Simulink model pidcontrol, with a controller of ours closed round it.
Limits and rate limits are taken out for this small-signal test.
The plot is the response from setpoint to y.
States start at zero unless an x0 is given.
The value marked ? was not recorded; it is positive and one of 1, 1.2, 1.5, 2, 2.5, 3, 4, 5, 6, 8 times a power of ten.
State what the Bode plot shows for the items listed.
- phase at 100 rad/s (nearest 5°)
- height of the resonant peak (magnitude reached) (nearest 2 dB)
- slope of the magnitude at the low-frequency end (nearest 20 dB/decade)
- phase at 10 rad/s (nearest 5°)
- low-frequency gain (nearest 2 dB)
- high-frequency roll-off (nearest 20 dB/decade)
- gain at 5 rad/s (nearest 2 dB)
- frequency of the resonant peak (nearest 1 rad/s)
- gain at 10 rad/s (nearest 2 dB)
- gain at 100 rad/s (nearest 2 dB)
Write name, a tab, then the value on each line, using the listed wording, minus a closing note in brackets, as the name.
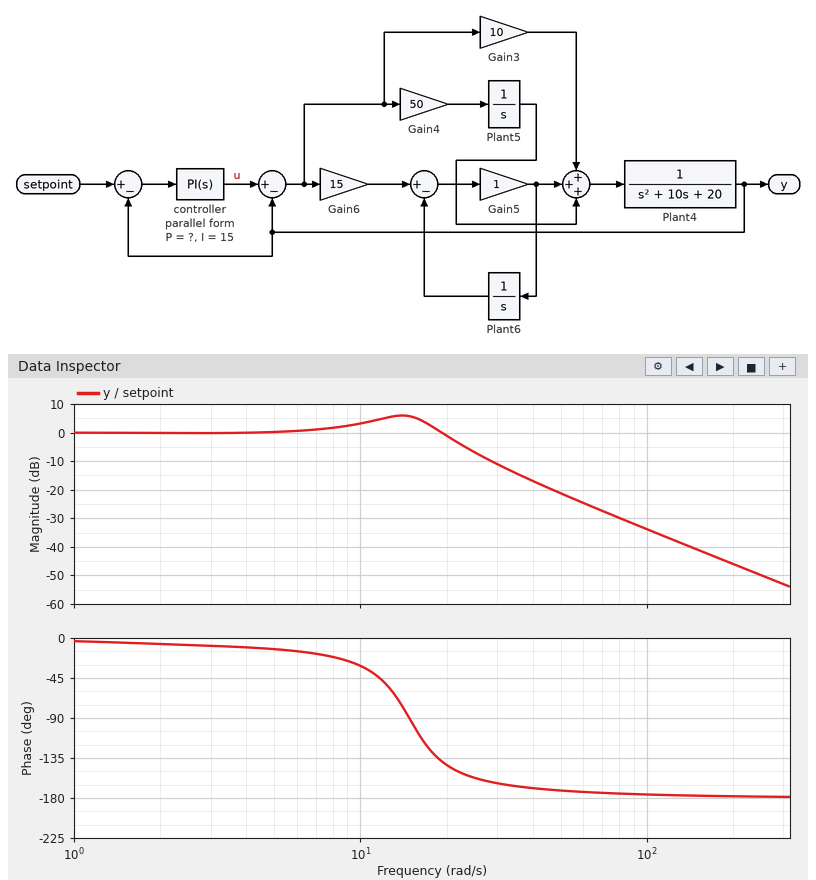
phase at 100 rad/s	-175°
height of the resonant peak (magnitude reached)	6 dB
slope of the magnitude at the low-frequency end	0 dB/decade
phase at 10 rad/s	-30°
low-frequency gain	0 dB
high-frequency roll-off	-40 dB/decade
gain at 5 rad/s	0 dB
frequency of the resonant peak	14 rad/s
gain at 10 rad/s	4 dB
gain at 100 rad/s	-34 dB
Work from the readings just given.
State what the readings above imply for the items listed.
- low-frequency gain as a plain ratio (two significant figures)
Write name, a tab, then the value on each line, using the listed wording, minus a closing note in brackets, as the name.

low-frequency gain as a plain ratio	1.0
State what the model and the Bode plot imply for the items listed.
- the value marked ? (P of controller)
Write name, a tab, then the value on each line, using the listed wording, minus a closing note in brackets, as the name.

the value marked ?	8
